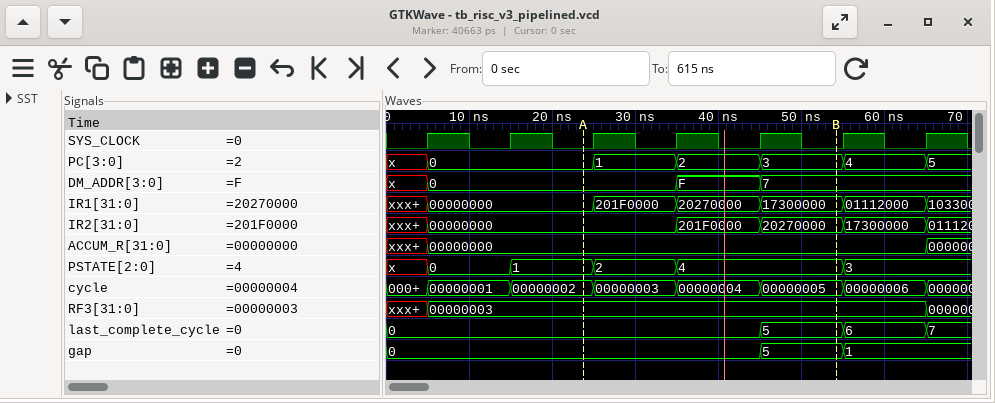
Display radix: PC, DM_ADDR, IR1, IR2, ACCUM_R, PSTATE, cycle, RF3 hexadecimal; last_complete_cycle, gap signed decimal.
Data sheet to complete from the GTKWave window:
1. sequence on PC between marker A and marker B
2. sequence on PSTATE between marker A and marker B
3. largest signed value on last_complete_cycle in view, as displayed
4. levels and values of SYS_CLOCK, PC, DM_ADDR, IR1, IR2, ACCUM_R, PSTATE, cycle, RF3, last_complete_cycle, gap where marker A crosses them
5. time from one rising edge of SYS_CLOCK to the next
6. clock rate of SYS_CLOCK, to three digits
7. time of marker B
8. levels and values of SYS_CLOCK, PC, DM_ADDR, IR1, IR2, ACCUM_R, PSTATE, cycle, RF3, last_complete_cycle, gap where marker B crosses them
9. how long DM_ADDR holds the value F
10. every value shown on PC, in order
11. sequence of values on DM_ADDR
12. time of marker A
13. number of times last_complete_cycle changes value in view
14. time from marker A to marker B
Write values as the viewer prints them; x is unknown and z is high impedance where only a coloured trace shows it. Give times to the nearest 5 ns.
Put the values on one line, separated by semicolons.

0, 1, 2, 3; 1, 2, 4; 7; SYS_CLOCK=0, PC=0, DM_ADDR=0, IR1=00000000, IR2=00000000, ACCUM_R=00000000, PSTATE=1, cycle=00000002, RF3=00000003, last_complete_cycle=0, gap=0; 10 ns; 100 MHz; 55 ns; SYS_CLOCK=0, PC=3, DM_ADDR=7, IR1=17300000, IR2=20270000, ACCUM_R=00000000, PSTATE=4, cycle=00000005, RF3=00000003, last_complete_cycle=5, gap=5; 10 ns; x, 0, 1, 2, 3, 4, 5; x, 0, F, 7; 25 ns; 3; 30 ns
